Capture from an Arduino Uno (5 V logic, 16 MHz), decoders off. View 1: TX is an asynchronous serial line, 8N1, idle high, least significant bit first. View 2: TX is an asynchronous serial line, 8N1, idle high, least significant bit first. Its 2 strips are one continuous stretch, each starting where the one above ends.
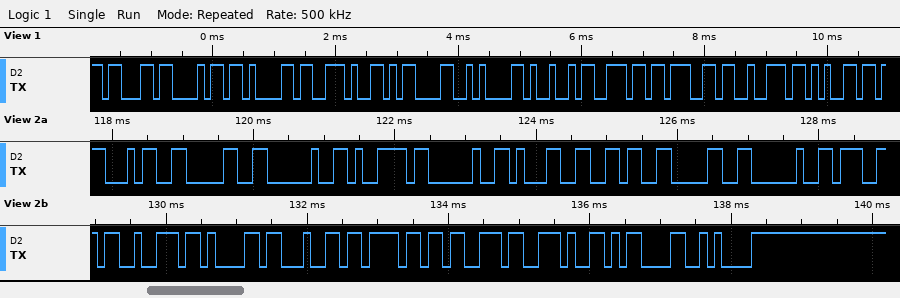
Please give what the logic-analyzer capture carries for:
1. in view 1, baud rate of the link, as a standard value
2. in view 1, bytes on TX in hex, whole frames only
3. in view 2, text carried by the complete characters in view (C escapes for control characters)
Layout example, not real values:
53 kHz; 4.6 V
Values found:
9600 baud; 63 68 61 2E 0D 0A 49 6E 67 72 65; "40 y 160 grados.\r\n"
